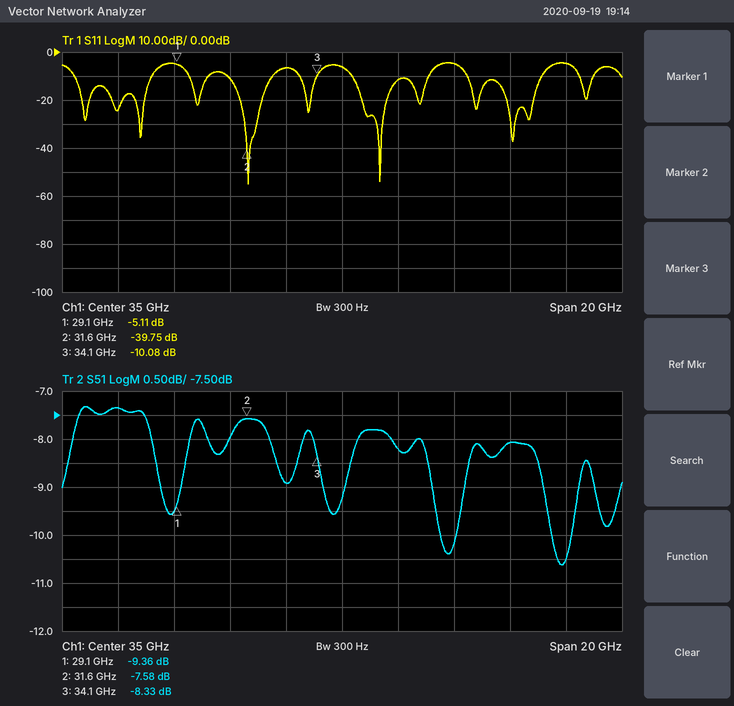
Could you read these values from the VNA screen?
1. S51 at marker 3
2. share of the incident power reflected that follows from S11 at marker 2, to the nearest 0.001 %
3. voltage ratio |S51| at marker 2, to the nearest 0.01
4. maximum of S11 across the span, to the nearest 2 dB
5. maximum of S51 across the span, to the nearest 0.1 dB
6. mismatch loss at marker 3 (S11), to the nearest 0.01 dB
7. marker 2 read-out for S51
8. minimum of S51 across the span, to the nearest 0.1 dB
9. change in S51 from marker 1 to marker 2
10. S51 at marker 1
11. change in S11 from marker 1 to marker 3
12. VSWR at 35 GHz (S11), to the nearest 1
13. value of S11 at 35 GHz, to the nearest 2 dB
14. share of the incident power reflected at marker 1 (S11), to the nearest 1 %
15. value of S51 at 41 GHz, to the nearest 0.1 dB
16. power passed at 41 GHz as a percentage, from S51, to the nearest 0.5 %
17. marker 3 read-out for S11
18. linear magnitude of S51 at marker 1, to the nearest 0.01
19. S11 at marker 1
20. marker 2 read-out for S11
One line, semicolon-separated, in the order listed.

-8.33 dB; 0.011 %; 0.42; -4 dB; -7.3 dB; 0.45 dB; -7.58 dB; -10.6 dB; 1.78 dB; -9.36 dB; -4.97 dB; 3; -6 dB; 31 %; -8.1 dB; 15.5 %; -10.08 dB; 0.34; -5.11 dB; -39.75 dB
